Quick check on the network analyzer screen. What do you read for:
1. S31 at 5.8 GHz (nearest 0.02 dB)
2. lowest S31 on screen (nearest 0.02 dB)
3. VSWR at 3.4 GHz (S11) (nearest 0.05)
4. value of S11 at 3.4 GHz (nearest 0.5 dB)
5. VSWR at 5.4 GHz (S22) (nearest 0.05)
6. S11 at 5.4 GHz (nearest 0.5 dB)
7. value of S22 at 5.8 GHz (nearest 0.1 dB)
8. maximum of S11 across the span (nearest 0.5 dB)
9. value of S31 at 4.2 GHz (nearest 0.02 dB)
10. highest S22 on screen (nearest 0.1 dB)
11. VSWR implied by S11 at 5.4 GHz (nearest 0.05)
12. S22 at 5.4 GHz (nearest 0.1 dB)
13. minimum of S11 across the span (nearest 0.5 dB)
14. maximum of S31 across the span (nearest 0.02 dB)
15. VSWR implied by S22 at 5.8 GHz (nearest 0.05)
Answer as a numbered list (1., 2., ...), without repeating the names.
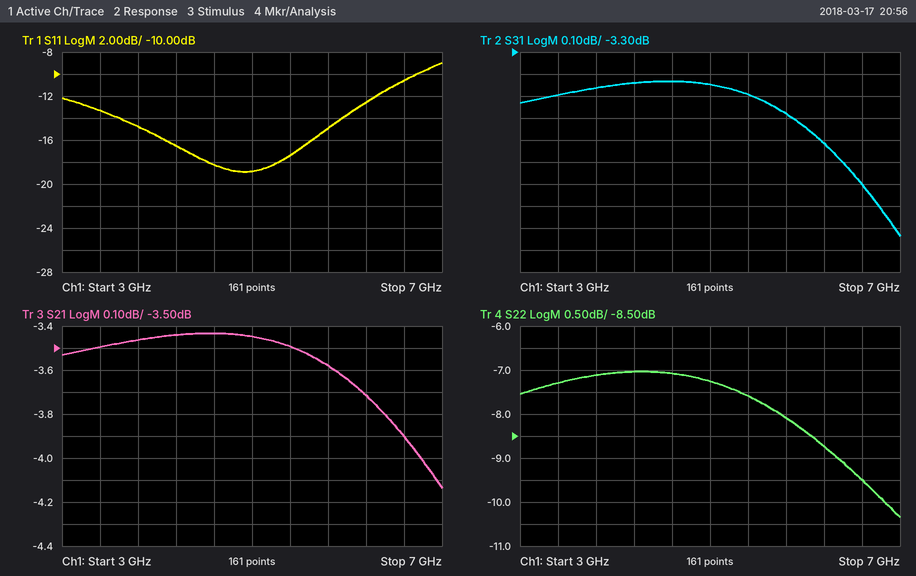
1. -3.58 dB
2. -4.14 dB
3. 1.55
4. -13.5 dB
5. 2.45
6. -17.5 dB
7. -8.1 dB
8. -9.0 dB
9. -3.44 dB
10. -7.0 dB
11. 1.30
12. -7.6 dB
13. -19.0 dB
14. -3.44 dB
15. 2.30
